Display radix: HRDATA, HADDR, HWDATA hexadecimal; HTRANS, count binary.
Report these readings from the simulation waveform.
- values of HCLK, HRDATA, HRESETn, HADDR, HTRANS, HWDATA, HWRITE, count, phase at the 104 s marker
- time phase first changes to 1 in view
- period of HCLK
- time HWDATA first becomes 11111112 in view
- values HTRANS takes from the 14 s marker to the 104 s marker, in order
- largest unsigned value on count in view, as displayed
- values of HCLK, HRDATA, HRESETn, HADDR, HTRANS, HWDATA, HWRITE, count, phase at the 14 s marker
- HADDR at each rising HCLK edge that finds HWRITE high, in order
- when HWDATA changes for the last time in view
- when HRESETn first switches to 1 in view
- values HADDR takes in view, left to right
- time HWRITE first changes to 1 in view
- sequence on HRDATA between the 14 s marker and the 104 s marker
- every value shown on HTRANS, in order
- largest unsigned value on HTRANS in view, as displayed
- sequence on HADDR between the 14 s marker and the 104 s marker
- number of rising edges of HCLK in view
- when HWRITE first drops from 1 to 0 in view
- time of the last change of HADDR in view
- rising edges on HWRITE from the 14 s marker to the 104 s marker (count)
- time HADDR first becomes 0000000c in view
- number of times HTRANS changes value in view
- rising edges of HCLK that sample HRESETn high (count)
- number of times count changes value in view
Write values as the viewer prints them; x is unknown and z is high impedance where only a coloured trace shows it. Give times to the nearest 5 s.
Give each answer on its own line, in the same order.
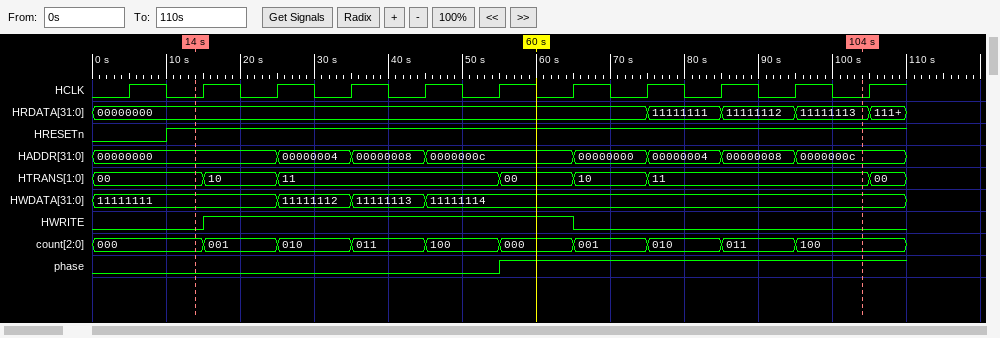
HCLK=0, HRDATA=11111113, HRESETn=1, HADDR=0000000c, HTRANS=11, HWDATA=11111114, HWRITE=0, count=100, phase=1
55 s
10 s
25 s
00, 10, 11, 00, 10, 11
100
HCLK=0, HRDATA=00000000, HRESETn=1, HADDR=00000000, HTRANS=00, HWDATA=11111111, HWRITE=0, count=000, phase=0
00000000, 00000004, 00000008, 0000000c, 0000000c
45 s
10 s
00000000, 00000004, 00000008, 0000000c, 00000000, 00000004, 00000008, 0000000c
15 s
00000000, 11111111, 11111112, 11111113
00, 10, 11, 00, 10, 11, 00
11
00000000, 00000004, 00000008, 0000000c, 00000000, 00000004, 00000008, 0000000c
11
65 s
95 s
1
45 s
6
10
9
